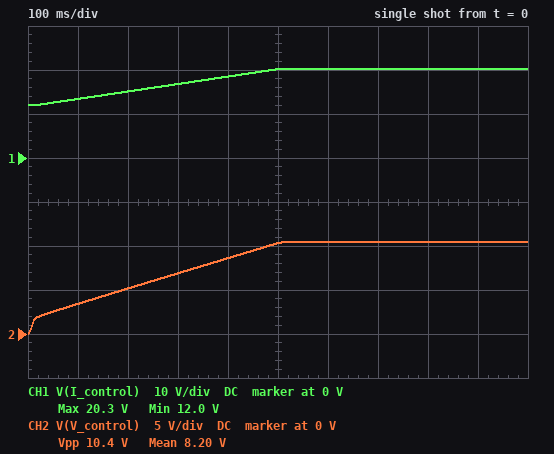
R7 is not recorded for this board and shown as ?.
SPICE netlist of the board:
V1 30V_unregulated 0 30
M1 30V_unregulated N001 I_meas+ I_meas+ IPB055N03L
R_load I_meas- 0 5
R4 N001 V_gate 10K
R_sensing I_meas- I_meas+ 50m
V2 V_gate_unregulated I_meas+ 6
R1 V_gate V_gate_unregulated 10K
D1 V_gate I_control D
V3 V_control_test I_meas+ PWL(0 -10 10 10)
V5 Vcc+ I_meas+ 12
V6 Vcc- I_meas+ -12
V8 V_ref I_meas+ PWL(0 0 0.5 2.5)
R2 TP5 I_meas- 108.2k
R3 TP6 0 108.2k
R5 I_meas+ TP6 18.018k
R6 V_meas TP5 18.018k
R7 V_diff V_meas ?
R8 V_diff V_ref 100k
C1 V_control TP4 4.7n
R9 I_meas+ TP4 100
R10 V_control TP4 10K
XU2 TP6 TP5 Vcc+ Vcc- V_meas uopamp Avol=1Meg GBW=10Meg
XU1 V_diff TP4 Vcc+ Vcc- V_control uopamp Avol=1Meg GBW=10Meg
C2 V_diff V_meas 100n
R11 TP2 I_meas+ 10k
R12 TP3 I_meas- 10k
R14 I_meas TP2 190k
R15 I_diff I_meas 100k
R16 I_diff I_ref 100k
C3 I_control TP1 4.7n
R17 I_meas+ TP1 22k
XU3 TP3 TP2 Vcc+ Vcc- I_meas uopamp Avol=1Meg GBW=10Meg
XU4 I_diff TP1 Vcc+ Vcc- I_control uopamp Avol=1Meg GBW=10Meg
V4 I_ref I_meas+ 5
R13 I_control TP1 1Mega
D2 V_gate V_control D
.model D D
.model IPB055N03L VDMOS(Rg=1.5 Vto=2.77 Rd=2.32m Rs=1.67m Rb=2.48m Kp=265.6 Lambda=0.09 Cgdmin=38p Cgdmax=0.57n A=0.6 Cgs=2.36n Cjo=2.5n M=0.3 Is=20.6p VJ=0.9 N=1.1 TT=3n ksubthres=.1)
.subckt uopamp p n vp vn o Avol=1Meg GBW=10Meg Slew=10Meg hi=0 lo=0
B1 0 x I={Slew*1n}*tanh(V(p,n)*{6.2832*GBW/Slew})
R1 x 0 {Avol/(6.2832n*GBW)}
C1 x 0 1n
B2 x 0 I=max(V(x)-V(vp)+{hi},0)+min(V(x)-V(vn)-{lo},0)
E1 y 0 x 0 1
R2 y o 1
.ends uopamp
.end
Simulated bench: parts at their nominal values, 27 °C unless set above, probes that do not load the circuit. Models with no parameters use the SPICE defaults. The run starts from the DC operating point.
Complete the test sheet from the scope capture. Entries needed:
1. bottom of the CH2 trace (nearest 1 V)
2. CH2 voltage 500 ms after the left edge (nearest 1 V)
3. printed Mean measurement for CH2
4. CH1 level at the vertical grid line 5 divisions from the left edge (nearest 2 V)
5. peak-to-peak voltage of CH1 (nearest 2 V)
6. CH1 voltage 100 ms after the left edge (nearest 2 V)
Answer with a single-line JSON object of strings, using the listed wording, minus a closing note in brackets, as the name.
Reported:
{"bottom of the CH2 trace": "0 V", "CH2 voltage 500 ms after the left edge": "10 V", "printed Mean measurement for CH2": "8.20 V", "CH1 level at the vertical grid line 5 divisions from the left edge": "20 V", "peak-to-peak voltage of CH1": "8 V", "CH1 voltage 100 ms after the left edge": "14 V"}
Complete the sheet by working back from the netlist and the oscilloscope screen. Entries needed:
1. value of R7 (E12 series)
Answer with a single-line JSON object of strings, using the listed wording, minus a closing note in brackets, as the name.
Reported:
{"value of R7": "56 kΩ"}
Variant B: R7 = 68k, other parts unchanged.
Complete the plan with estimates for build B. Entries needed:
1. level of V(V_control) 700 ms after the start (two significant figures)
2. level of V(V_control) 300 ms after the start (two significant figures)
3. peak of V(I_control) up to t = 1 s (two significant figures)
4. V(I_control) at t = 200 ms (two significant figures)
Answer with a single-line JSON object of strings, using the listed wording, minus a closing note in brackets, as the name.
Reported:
{"level of V(V_control) 700 ms after the start": "12 V", "level of V(V_control) 300 ms after the start": "7.9 V", "peak of V(I_control) up to t = 1 s": "22 V", "V(I_control) at t = 200 ms": "16 V"}
